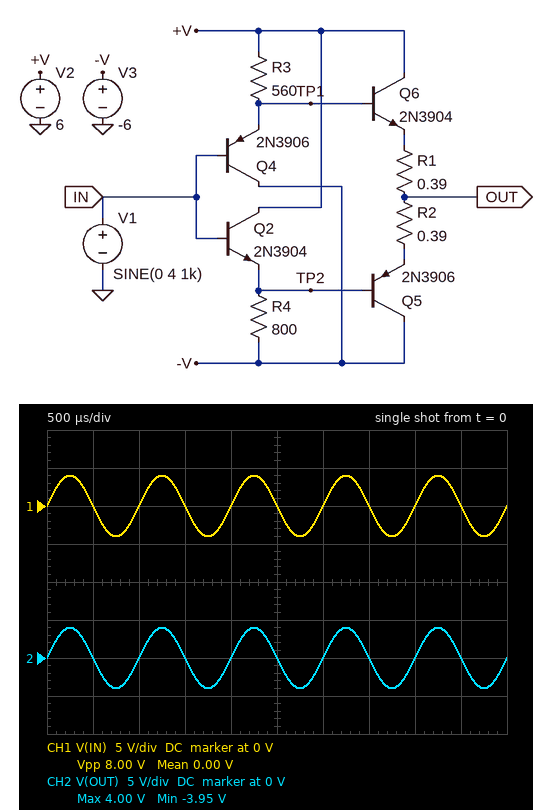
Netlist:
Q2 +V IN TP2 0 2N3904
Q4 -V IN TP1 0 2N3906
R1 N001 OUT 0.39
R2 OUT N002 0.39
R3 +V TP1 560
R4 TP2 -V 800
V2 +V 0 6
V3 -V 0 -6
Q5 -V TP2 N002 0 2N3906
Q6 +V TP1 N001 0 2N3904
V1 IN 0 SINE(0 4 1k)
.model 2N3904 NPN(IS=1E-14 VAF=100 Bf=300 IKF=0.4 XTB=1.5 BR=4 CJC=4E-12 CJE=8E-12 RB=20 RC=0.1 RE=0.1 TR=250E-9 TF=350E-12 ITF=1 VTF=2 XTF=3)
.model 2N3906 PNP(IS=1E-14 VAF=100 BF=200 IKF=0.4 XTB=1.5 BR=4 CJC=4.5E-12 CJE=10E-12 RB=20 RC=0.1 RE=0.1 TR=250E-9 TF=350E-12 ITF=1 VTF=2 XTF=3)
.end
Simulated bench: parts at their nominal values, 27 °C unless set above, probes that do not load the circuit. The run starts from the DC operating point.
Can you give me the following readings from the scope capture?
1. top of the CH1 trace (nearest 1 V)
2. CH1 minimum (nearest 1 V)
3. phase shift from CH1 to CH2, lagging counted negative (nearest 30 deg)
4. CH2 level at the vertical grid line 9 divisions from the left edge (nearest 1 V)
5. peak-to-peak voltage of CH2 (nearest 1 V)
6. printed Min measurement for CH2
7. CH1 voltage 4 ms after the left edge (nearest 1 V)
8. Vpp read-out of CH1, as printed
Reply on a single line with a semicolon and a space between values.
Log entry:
4 V; -4 V; 0 deg; 0 V; 8 V; -3.95 V; 0 V; 8.00 V
